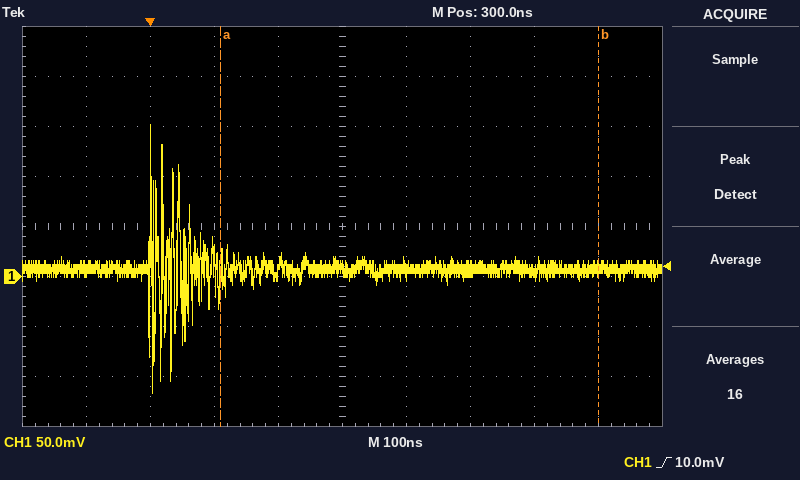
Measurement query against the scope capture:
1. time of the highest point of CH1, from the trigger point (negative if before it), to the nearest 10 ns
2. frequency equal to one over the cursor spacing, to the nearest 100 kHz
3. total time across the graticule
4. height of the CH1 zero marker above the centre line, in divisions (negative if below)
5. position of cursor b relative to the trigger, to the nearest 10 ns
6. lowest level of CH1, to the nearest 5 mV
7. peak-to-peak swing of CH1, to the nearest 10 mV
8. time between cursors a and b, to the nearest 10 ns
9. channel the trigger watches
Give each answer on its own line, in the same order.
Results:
0 ns
1.7 MHz
1 µs
-1.0 div
+700 ns
-115 mV
270 mV
590 ns
CH1
